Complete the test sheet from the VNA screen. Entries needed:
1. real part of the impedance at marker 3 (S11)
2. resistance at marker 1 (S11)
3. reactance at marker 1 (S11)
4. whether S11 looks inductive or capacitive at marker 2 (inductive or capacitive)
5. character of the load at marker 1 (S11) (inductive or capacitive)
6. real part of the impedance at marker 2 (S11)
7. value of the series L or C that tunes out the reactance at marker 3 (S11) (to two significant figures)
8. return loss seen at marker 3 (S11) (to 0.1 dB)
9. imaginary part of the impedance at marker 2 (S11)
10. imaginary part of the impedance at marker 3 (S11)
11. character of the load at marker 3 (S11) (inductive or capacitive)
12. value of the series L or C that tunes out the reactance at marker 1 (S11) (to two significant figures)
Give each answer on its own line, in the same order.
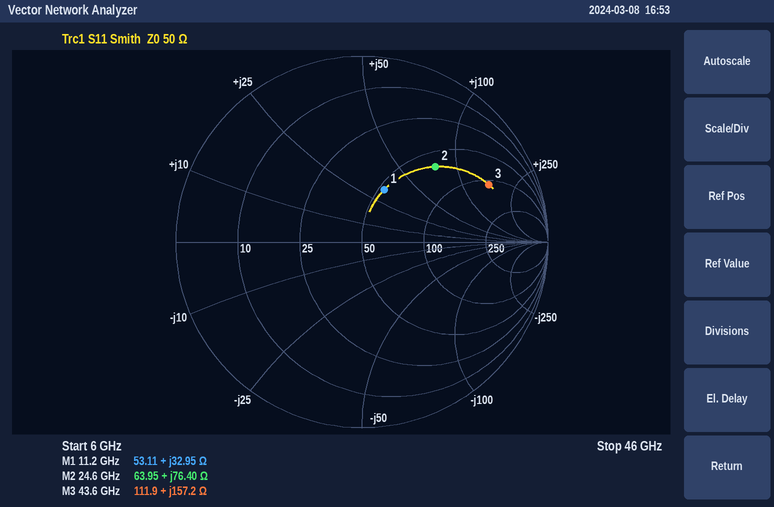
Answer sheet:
111.9 Ω
53.11 Ω
+32.95 Ω
inductive
inductive
63.95 Ω
23 fF
2.5 dB
+76.40 Ω
+157.2 Ω
inductive
430 fF
